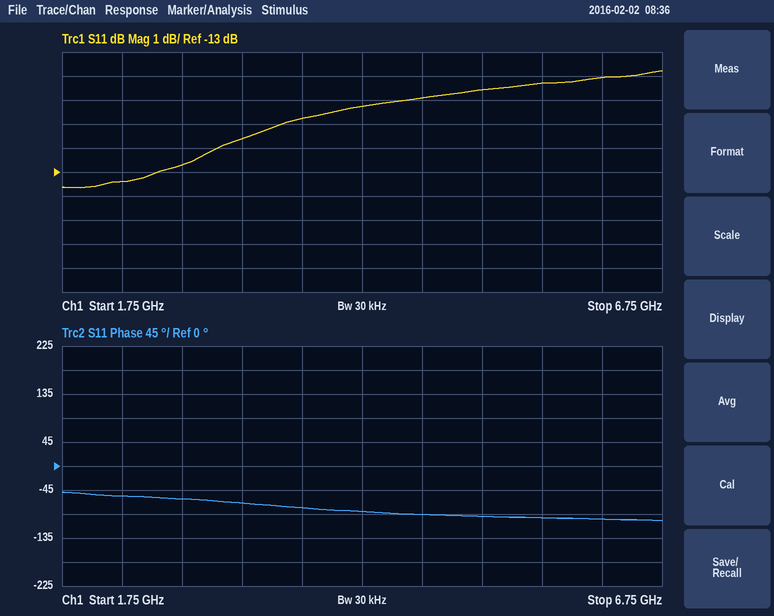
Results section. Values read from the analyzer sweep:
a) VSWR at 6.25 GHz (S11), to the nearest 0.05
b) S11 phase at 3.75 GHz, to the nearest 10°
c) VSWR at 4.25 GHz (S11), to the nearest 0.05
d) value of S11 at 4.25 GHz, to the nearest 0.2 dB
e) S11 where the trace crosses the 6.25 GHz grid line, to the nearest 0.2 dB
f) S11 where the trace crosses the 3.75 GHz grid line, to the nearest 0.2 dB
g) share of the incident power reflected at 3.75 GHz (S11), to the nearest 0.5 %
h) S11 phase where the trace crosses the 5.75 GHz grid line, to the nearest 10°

2.10
-80°
1.90
-10.2 dB
-9.0 dB
-10.8 dB
8.5 %
-100°
